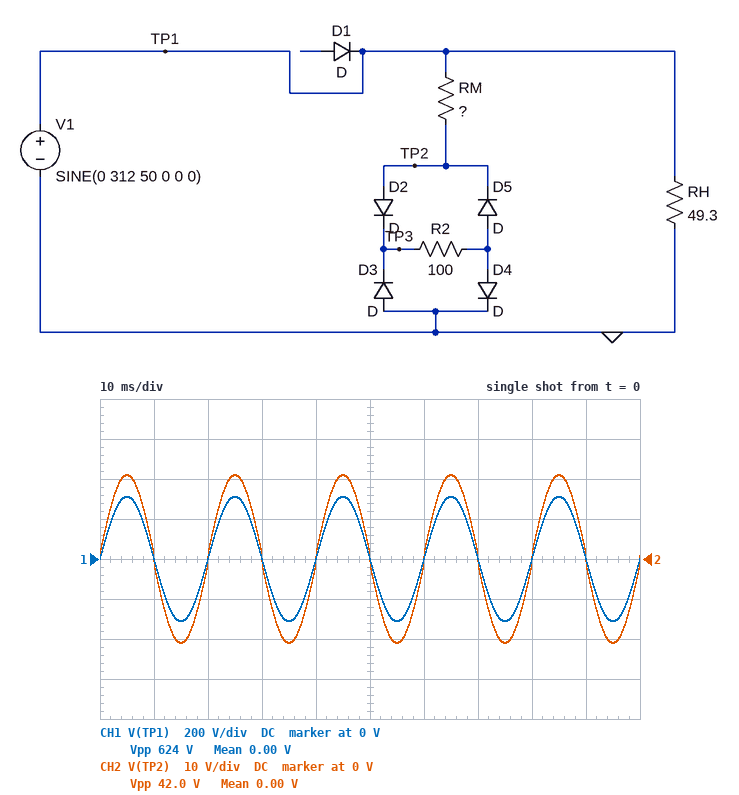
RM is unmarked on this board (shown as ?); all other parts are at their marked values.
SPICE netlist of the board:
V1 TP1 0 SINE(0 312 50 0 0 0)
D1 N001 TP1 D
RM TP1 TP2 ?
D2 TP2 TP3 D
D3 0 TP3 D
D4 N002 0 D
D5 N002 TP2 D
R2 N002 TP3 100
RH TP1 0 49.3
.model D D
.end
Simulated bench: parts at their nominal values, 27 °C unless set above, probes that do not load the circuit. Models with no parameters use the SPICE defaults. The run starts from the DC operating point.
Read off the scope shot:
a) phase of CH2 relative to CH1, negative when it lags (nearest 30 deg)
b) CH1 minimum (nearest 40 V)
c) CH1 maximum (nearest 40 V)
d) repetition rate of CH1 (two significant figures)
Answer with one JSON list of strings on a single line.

["0 deg", "-320 V", "320 V", "50 Hz"]
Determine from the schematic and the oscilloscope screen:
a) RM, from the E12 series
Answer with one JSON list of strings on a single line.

["1.5 kΩ"]
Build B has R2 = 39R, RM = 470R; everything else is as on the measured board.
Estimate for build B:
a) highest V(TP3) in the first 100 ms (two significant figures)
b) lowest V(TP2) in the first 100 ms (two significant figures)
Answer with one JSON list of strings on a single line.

["25 V", "-25 V"]
